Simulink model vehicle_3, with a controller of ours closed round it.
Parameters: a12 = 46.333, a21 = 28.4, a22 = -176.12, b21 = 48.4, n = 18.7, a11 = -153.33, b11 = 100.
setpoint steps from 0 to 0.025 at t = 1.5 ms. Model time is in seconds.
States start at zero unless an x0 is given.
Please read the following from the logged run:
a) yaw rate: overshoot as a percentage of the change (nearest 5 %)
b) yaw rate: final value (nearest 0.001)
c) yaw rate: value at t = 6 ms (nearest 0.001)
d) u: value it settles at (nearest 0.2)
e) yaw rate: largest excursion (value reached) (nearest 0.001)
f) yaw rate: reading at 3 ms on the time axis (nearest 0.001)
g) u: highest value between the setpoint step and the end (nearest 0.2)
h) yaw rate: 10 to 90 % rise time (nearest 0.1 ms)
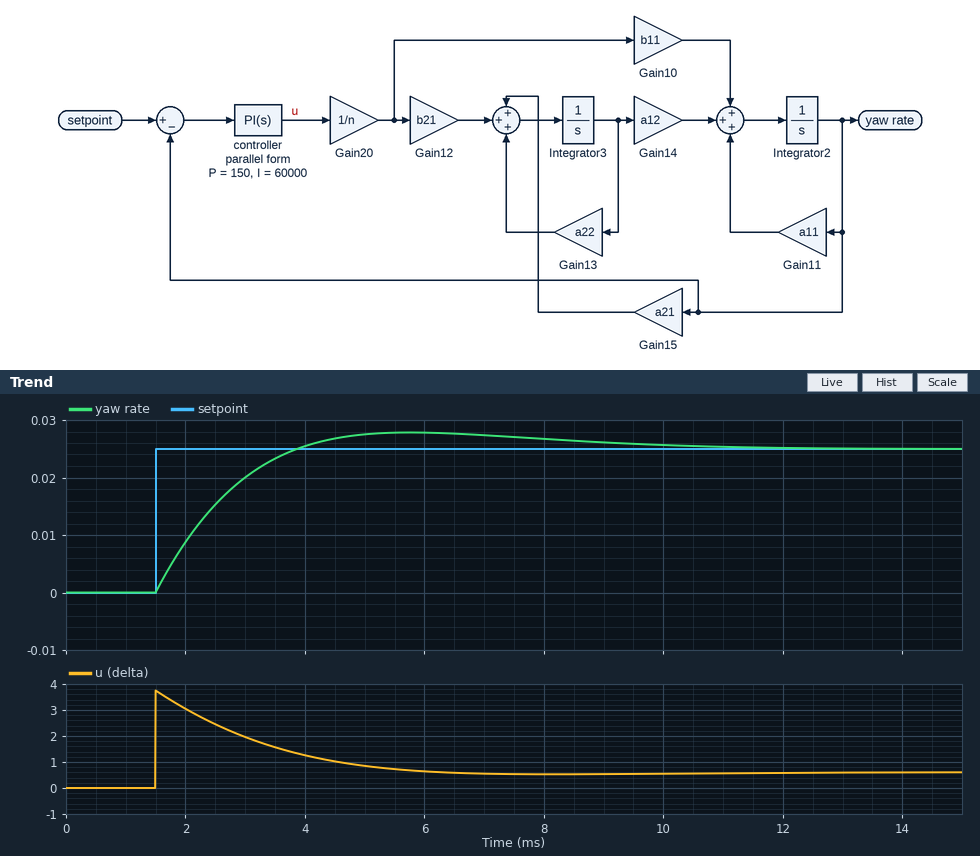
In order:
10 %
0.025
0.028
0.6
0.028
0.020
3.8
1.7 ms
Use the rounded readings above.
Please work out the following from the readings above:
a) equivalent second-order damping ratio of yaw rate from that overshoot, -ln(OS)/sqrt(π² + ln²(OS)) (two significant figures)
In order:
0.59
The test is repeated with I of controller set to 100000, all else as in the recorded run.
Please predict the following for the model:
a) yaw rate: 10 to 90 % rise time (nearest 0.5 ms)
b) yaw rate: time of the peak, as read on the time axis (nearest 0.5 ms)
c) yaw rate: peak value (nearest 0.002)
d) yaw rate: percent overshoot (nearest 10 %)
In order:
1.5 ms
5.0 ms
0.030
20 %
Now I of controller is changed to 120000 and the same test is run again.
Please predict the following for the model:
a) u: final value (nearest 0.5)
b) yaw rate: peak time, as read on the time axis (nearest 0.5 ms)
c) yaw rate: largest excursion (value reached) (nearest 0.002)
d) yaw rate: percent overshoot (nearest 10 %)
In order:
0.5
4.5 ms
0.030
20 %
